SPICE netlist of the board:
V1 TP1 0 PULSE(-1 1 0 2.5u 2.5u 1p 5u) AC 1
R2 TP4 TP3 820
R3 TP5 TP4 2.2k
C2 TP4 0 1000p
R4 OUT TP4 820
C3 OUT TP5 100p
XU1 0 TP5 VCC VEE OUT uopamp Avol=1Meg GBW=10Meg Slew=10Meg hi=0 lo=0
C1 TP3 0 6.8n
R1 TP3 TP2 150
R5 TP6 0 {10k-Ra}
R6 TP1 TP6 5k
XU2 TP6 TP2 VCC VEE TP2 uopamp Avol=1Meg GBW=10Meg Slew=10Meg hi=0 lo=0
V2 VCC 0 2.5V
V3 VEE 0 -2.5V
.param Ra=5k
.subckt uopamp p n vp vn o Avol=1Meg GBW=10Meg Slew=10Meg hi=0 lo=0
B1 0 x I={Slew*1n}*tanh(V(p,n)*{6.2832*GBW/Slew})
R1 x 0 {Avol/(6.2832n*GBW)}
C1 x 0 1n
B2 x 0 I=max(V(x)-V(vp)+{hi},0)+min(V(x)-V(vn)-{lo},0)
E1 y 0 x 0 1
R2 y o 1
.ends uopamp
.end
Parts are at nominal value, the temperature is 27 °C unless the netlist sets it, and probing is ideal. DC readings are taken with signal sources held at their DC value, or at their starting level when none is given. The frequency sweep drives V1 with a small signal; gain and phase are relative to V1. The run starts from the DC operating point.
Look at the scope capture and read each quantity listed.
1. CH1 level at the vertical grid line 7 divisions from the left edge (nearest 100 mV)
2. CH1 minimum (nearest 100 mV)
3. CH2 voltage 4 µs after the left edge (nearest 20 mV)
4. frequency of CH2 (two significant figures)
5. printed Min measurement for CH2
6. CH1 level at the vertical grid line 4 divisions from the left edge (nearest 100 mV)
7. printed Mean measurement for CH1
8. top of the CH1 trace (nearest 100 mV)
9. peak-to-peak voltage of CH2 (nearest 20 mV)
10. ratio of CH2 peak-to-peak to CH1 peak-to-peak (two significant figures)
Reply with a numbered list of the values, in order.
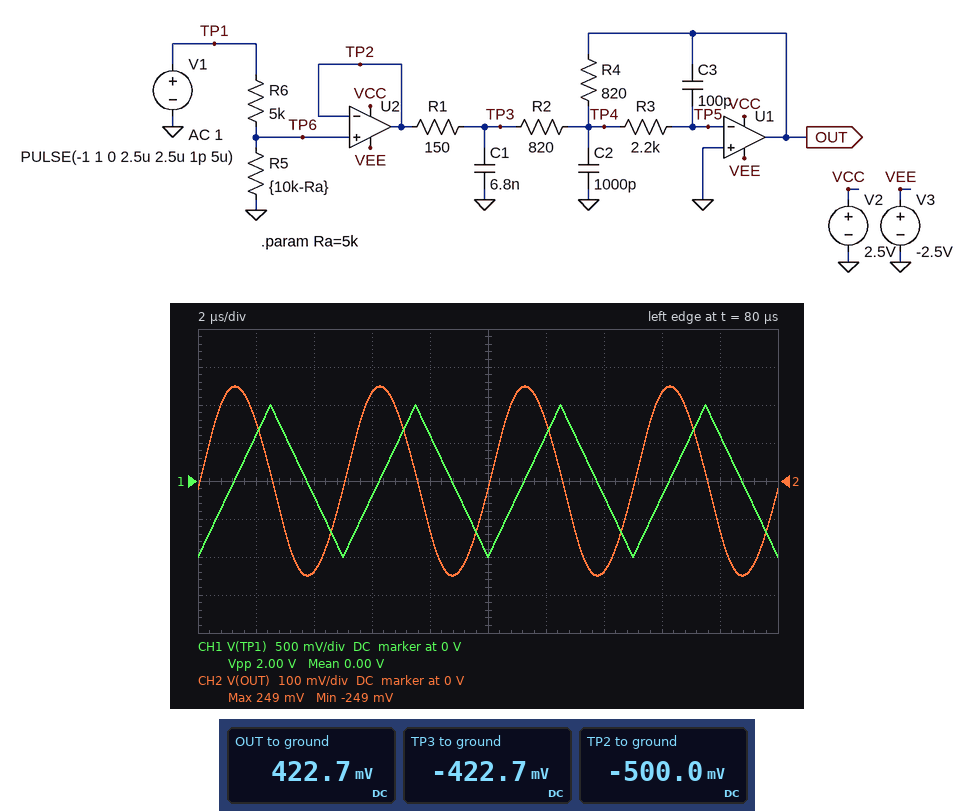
1. -200 mV
2. -1.0 V
3. -240 mV
4. 200 kHz
5. -249 mV
6. 600 mV
7. 0.00 V
8. 1.0 V
9. 500 mV
10. 0.25
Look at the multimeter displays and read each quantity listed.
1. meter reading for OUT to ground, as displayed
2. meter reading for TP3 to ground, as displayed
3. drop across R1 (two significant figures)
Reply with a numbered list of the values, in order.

1. 422.7 mV
2. -422.7 mV
3. 77 mV
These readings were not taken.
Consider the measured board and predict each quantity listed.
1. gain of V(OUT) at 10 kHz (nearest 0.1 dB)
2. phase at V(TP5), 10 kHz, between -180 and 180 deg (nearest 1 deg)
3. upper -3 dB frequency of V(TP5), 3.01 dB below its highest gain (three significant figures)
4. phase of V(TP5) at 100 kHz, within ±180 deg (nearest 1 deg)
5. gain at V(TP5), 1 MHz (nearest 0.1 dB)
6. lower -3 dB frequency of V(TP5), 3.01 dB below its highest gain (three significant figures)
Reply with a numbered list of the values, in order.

1. -7.5 dB
2. 85 deg
3. 438 kHz
4. 41 deg
5. -59.9 dB
6. 127 kHz
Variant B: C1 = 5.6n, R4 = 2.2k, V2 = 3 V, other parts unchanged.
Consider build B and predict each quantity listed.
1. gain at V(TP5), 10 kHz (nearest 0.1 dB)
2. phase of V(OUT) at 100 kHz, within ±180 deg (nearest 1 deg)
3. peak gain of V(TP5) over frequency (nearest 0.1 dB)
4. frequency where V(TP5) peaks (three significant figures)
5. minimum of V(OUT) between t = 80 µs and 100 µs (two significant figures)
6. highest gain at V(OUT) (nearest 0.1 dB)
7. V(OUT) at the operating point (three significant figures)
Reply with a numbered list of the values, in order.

1. -58.9 dB
2. 116 deg
3. -37.4 dB
4. 173 kHz
5. -530 mV
6. 1.1 dB
7. 1.13 V
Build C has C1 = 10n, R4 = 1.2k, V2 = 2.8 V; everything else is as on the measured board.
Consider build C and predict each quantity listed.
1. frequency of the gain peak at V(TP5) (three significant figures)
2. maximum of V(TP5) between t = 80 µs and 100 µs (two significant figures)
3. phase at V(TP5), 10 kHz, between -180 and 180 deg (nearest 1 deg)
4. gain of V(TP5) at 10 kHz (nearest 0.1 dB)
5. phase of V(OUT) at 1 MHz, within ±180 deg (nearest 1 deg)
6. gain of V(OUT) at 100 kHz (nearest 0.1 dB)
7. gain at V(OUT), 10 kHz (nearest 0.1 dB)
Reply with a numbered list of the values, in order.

1. 202 kHz
2. 5.5 mV
3. 83 deg
4. -64.2 dB
5. -71 deg
6. -6.0 dB
7. -4.2 dB
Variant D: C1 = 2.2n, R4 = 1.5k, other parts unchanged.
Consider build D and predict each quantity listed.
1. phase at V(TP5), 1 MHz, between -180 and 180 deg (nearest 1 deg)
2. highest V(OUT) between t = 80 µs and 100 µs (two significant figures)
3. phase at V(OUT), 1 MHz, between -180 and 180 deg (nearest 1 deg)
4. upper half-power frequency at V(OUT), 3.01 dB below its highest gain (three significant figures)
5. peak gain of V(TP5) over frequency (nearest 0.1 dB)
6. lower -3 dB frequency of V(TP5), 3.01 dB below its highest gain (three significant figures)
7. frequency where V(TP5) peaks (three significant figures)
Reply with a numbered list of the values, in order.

1. -141 deg
2. 580 mV
3. -51 deg
4. 268 kHz
5. -36.4 dB
6. 137 kHz
7. 244 kHz
